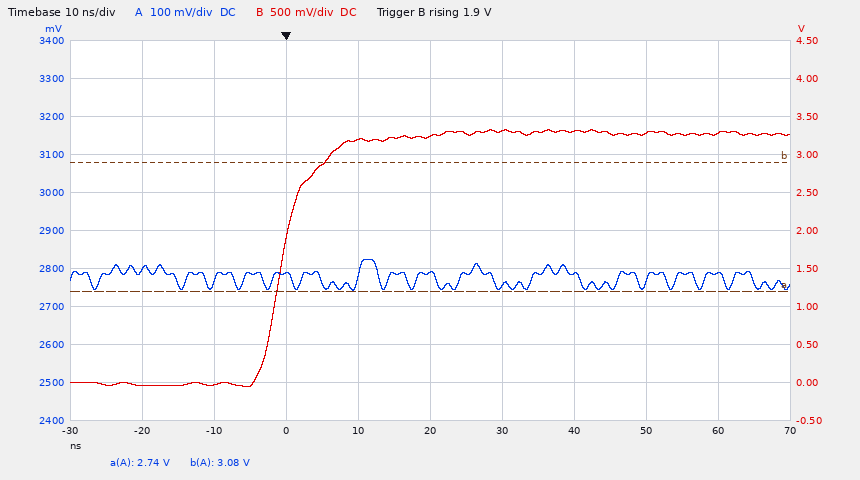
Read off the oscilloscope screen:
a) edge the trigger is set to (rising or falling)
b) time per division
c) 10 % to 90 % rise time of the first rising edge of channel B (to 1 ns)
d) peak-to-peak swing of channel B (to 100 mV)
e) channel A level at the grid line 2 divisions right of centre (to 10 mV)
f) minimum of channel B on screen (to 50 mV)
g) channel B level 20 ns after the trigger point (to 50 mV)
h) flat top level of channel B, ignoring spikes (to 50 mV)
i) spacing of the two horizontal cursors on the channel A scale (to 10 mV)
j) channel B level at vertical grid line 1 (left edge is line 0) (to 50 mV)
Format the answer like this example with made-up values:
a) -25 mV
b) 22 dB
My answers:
a) rising
b) 10 ns
c) 9 ns
d) 3.40 V
e) 2.79 V
f) -50 mV
g) 3.25 V
h) 3.30 V
i) 340 mV
j) -50 mV
